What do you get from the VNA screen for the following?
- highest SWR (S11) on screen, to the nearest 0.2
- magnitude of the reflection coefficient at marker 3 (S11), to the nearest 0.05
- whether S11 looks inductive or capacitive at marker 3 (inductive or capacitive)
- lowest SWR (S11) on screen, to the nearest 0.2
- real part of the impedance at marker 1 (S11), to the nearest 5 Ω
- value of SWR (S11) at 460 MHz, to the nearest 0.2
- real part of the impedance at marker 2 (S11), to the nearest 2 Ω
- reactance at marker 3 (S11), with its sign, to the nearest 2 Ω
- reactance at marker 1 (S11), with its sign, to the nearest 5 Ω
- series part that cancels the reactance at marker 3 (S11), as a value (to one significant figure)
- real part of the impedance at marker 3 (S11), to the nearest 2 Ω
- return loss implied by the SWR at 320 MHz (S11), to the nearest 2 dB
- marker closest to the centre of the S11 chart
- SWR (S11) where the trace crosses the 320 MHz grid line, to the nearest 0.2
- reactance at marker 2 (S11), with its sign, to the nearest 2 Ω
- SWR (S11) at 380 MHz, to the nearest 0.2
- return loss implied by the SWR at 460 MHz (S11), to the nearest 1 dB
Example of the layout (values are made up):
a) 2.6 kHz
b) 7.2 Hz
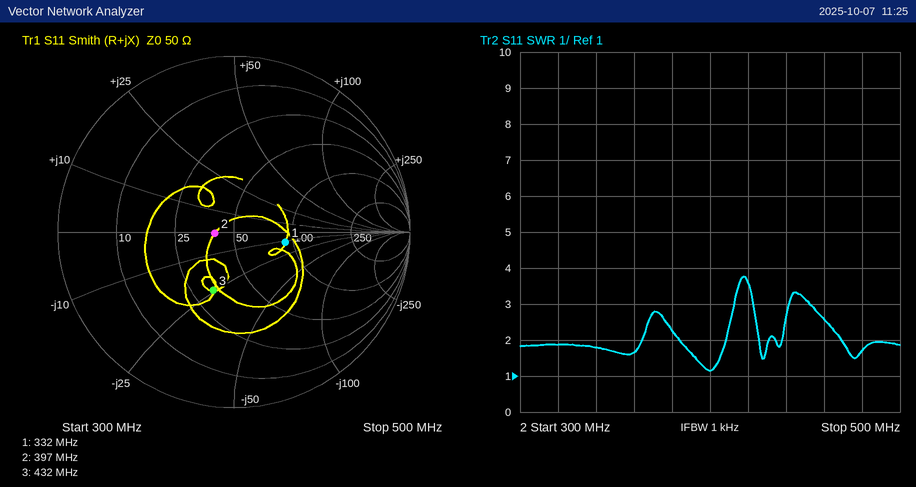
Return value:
a) 3.8
b) 0.35
c) capacitive
d) 1.2
e) 90 Ω
f) 2.6
g) 40 Ω
h) -24 Ω
i) -10 Ω
j) 9 nH
k) 32 Ω
l) 10 dB
m) marker 2
n) 1.8
o) 0 Ω
p) 2.2
q) 7 dB
